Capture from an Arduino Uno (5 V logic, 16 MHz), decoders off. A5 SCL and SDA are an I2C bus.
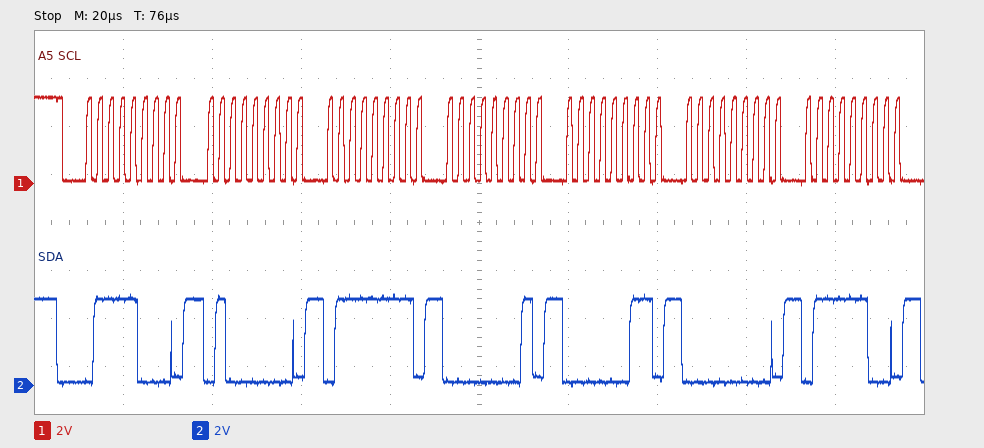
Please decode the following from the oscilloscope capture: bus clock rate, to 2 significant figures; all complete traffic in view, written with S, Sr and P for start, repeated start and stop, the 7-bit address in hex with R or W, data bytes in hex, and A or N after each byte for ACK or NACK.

400 kHz
S 3CW A 40 A 7F A 01 A 03 A 00 A 7C A
